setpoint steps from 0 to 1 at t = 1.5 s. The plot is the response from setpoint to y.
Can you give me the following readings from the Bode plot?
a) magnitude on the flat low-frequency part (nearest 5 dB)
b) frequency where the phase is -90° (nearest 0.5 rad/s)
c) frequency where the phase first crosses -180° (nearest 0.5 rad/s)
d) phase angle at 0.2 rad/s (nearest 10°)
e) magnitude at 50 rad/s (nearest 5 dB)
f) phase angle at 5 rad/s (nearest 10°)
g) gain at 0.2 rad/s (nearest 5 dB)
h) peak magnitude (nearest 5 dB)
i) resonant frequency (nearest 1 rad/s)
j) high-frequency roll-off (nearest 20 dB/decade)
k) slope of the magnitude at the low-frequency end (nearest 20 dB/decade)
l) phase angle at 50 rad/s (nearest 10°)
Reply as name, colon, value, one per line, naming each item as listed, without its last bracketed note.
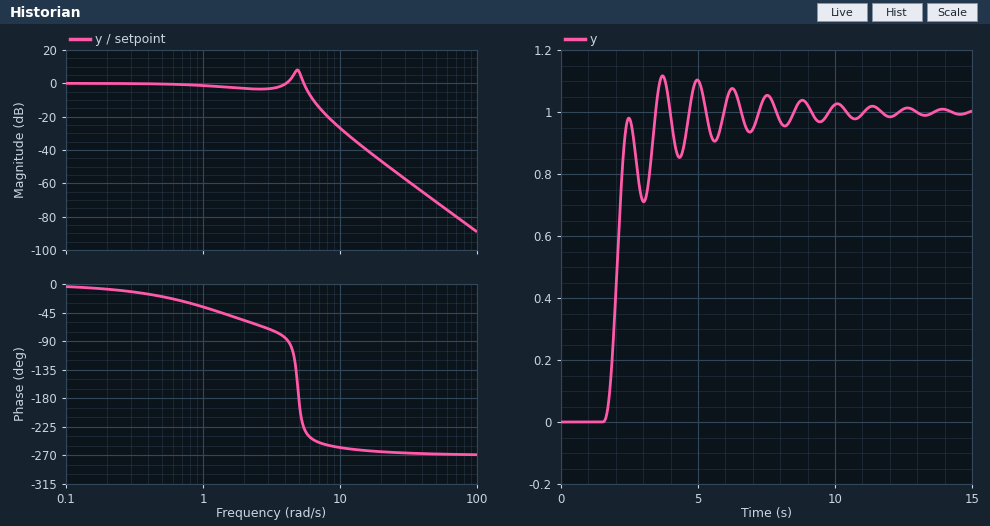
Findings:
magnitude on the flat low-frequency part: 0 dB
frequency where the phase is -90°: 4.0 rad/s
frequency where the phase first crosses -180°: 5.0 rad/s
phase angle at 0.2 rad/s: -10°
magnitude at 50 rad/s: -70 dB
phase angle at 5 rad/s: -180°
gain at 0.2 rad/s: 0 dB
peak magnitude: 10 dB
resonant frequency: 5 rad/s
high-frequency roll-off: -60 dB/decade
slope of the magnitude at the low-frequency end: 0 dB/decade
phase angle at 50 rad/s: -270°
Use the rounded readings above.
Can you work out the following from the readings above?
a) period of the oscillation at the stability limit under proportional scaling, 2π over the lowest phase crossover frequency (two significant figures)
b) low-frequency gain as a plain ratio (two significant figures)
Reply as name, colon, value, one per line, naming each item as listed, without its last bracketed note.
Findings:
period of the oscillation at the stability limit under proportional scaling, 2π over the lowest phase crossover frequency: 1.3 s
low-frequency gain as a plain ratio: 1.0
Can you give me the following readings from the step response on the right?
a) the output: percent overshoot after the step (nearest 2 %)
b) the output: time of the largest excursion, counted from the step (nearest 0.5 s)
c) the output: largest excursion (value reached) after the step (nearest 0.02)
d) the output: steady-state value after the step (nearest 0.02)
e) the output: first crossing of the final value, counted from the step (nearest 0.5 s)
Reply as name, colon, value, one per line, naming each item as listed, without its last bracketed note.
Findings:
the output: percent overshoot after the step: 12 %
the output: time of the largest excursion, counted from the step: 2.0 s
the output: largest excursion (value reached) after the step: 1.12
the output: steady-state value after the step: 1.00
the output: first crossing of the final value, counted from the step: 2.0 s
